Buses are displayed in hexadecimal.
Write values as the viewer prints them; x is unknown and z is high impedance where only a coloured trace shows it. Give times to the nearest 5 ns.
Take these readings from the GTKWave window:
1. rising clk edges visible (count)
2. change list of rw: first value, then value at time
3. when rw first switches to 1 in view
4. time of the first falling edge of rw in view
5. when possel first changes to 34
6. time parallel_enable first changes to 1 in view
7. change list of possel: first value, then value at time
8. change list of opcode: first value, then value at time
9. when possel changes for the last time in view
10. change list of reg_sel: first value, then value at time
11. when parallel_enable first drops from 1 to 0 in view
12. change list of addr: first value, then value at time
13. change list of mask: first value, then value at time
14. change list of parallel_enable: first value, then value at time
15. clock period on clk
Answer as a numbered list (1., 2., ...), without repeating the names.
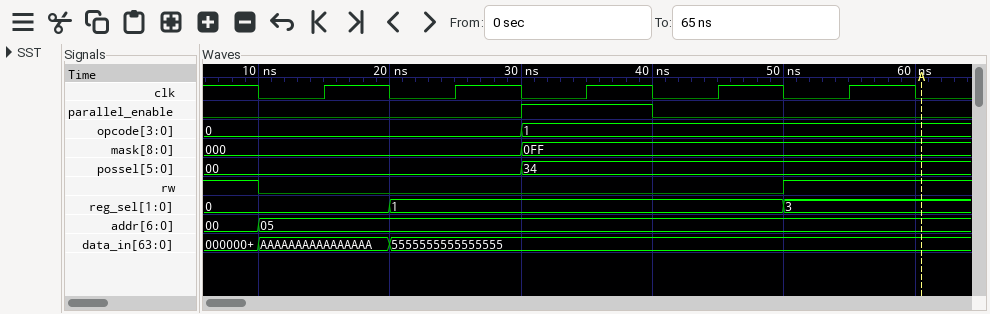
1. 5
2. 1, 0 at 10 ns, 1 at 50 ns
3. 50 ns
4. 10 ns
5. 30 ns
6. 30 ns
7. 00, 34 at 30 ns
8. 0, 1 at 30 ns
9. 30 ns
10. 0, 1 at 20 ns, 3 at 50 ns
11. 40 ns
12. 00, 05 at 10 ns
13. 000, 0FF at 30 ns
14. 0, 1 at 30 ns, 0 at 40 ns
15. 10 ns
